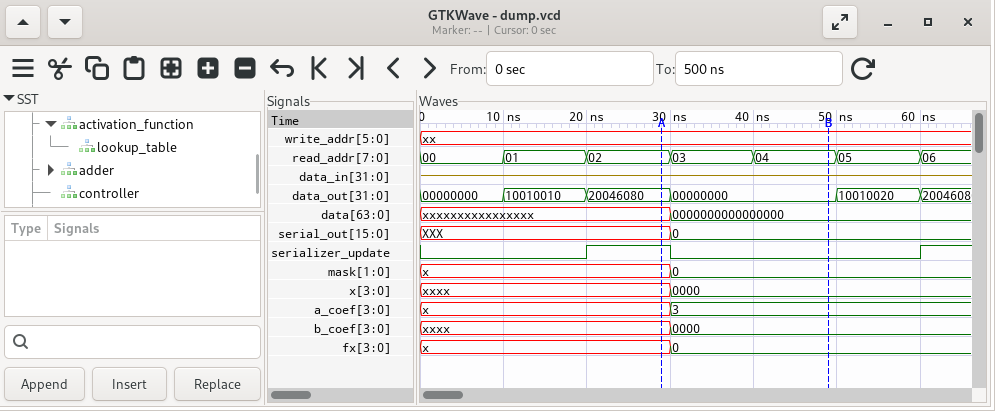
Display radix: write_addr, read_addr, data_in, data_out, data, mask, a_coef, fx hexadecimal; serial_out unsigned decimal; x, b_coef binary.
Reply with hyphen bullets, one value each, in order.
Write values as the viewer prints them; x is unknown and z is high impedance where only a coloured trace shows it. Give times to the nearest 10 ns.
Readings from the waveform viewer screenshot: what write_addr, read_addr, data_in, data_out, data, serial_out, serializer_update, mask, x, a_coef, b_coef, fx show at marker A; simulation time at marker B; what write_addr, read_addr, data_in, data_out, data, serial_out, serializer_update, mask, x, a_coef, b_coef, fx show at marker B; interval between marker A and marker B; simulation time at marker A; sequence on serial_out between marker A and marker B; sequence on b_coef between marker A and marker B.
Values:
- write_addr=xx, read_addr=02, data_in=z, data_out=20046080, data=xxxxxxxxxxxxxxxx, serial_out=XXX, serializer_update=1, mask=x, x=xxxx, a_coef=x, b_coef=xxxx, fx=x
- 50 ns
- write_addr=xx, read_addr=04, data_in=z, data_out=00000000, data=0000000000000000, serial_out=0, serializer_update=0, mask=0, x=0000, a_coef=3, b_coef=0000, fx=0
- 20 ns
- 30 ns
- XXX, 0
- xxxx, 0000
